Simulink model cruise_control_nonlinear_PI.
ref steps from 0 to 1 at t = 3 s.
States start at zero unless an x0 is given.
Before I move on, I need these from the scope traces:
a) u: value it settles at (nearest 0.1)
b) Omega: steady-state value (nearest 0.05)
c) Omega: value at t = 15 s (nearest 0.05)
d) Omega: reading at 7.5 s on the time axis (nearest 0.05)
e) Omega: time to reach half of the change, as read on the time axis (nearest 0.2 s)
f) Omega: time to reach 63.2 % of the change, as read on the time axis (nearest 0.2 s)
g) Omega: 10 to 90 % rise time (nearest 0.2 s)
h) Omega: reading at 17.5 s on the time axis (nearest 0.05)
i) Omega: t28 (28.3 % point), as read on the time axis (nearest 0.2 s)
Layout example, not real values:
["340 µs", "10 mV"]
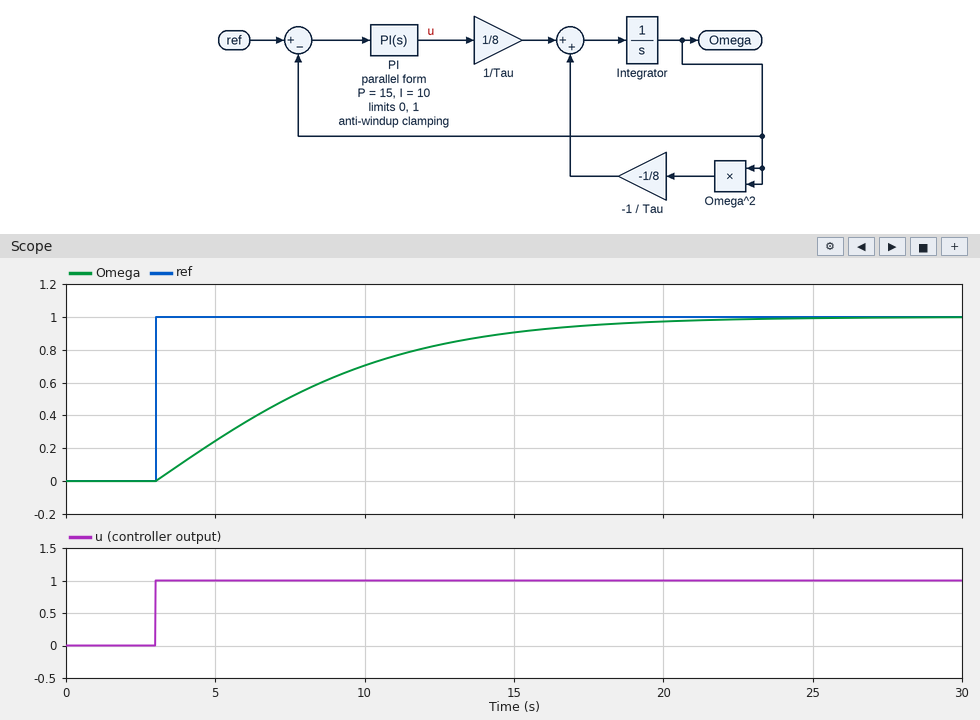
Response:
["1.0", "1.00", "0.90", "0.50", "7.4 s", "9.0 s", "11.0 s", "0.95", "5.4 s"]
